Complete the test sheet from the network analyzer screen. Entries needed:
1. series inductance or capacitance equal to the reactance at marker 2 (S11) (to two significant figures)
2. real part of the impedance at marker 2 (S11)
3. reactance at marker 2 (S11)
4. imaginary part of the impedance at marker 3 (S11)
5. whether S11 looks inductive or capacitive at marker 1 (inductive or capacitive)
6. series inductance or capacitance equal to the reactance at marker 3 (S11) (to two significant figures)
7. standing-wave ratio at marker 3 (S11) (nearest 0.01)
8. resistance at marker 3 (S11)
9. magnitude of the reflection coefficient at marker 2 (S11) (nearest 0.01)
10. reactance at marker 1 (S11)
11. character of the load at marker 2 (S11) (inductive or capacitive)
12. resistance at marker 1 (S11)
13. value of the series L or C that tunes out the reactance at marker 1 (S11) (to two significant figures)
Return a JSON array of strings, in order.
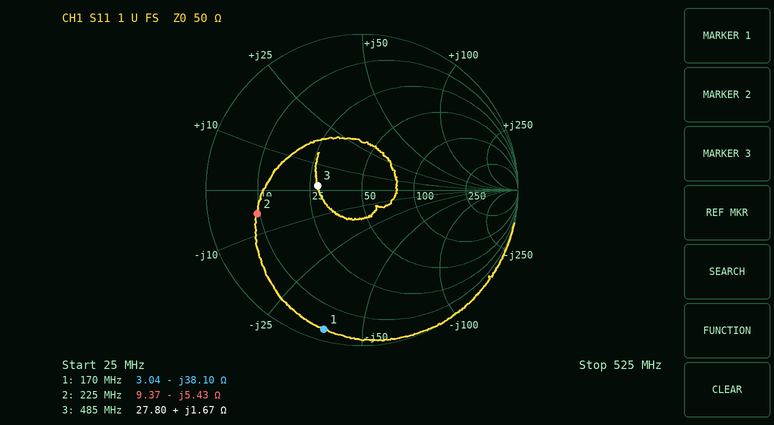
["130 pF", "9.37 Ω", "-5.43 Ω", "+1.67 Ω", "capacitive", "550 pH", "1.80", "27.80 Ω", "0.69", "-38.10 Ω", "capacitive", "3.04 Ω", "36 nH"]
